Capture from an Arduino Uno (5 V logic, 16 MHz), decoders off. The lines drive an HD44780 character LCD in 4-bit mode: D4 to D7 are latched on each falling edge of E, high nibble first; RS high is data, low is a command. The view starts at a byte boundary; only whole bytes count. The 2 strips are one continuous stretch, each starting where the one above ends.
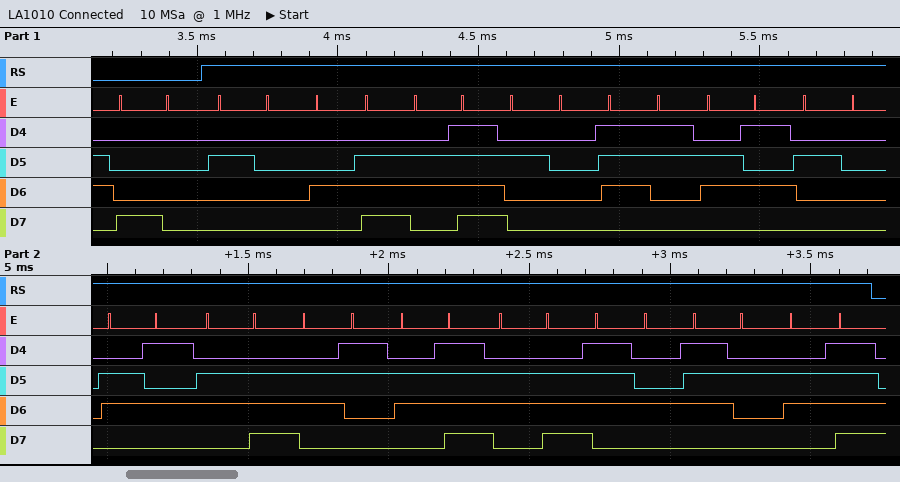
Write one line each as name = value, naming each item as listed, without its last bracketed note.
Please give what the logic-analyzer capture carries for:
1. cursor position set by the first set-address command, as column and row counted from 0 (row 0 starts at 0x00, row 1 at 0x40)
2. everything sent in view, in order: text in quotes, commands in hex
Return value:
cursor position set by the first set-address command, as column and row counted from 0 = column 0, row 0
everything sent in view, in order: text in quotes, commands in hex = 0x80 " No se encontro"
